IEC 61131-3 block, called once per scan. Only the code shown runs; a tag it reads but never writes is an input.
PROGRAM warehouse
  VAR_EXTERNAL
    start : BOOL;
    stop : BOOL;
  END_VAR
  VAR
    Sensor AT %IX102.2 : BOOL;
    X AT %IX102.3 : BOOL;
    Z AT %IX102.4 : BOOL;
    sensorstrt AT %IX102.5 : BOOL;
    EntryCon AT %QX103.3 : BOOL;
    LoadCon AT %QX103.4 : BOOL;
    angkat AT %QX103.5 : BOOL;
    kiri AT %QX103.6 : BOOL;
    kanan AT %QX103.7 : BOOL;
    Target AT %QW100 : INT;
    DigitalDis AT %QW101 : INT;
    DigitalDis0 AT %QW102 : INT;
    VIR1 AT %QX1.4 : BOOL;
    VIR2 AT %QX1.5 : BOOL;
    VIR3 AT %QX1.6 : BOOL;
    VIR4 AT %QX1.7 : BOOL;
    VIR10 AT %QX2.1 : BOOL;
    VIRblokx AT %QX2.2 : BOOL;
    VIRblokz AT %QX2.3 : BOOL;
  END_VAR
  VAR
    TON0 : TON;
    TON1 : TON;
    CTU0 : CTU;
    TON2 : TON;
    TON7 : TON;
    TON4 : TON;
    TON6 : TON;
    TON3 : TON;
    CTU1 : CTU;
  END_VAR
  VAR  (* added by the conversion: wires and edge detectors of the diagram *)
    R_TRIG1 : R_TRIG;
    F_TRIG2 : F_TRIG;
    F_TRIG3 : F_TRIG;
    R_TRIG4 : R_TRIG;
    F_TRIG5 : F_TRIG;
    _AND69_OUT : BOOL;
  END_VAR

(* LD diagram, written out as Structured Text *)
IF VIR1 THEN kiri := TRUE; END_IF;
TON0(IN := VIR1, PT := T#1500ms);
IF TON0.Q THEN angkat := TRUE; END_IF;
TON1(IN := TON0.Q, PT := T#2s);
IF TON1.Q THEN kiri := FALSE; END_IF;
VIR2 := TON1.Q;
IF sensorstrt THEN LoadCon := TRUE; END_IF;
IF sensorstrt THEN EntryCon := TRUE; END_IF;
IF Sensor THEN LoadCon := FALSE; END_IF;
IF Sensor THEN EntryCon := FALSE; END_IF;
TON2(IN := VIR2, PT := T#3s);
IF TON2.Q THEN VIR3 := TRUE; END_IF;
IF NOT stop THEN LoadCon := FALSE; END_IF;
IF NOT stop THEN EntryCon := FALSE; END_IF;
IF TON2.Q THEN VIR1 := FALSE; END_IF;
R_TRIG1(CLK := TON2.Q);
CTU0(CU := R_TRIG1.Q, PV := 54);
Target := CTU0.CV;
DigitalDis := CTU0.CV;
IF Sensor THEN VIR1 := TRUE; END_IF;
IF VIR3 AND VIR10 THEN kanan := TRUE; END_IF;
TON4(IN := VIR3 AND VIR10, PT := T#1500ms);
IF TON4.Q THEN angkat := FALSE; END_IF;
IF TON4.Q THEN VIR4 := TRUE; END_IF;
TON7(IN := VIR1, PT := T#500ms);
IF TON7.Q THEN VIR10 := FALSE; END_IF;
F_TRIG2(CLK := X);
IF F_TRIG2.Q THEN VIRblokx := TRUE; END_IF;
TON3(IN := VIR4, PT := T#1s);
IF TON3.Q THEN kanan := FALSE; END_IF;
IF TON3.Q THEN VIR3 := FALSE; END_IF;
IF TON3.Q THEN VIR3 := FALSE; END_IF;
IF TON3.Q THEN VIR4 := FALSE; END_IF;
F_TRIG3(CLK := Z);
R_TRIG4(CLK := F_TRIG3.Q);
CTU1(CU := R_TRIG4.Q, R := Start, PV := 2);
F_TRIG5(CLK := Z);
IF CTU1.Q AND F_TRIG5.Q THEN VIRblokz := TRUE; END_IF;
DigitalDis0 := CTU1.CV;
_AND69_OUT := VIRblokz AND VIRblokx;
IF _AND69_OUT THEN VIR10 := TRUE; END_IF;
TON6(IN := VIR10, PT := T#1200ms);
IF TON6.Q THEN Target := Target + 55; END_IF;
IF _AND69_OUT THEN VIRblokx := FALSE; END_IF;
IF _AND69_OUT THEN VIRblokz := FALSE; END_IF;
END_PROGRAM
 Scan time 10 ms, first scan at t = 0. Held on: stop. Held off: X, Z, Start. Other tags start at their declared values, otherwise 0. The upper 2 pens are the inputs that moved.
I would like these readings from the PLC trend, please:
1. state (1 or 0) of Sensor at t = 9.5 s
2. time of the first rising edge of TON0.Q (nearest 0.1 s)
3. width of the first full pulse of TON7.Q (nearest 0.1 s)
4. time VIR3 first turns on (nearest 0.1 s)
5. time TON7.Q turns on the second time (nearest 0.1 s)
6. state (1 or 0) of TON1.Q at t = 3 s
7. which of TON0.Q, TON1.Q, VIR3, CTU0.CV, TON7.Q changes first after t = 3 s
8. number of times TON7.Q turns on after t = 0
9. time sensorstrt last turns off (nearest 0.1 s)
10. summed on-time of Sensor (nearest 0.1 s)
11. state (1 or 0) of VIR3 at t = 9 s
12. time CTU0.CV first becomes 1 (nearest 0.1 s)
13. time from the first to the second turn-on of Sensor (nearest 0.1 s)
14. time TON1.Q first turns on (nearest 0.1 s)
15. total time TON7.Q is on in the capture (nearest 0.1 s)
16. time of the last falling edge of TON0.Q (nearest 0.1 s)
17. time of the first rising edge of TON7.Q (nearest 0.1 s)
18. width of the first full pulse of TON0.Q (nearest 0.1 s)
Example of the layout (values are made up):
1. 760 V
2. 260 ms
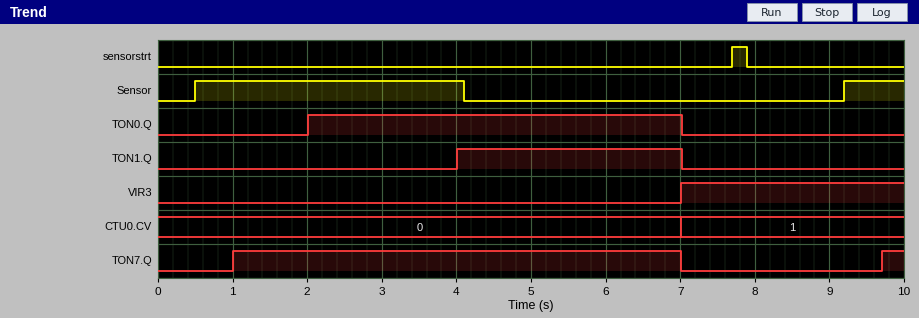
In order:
1. 1
2. 2.0 s
3. 6.0 s
4. 7.0 s
5. 9.7 s
6. 0
7. TON1.Q
8. 2
9. 7.9 s
10. 4.4 s
11. 1
12. 7.0 s
13. 8.7 s
14. 4.0 s
15. 6.3 s
16. 7.0 s
17. 1.0 s
18. 5.0 s
